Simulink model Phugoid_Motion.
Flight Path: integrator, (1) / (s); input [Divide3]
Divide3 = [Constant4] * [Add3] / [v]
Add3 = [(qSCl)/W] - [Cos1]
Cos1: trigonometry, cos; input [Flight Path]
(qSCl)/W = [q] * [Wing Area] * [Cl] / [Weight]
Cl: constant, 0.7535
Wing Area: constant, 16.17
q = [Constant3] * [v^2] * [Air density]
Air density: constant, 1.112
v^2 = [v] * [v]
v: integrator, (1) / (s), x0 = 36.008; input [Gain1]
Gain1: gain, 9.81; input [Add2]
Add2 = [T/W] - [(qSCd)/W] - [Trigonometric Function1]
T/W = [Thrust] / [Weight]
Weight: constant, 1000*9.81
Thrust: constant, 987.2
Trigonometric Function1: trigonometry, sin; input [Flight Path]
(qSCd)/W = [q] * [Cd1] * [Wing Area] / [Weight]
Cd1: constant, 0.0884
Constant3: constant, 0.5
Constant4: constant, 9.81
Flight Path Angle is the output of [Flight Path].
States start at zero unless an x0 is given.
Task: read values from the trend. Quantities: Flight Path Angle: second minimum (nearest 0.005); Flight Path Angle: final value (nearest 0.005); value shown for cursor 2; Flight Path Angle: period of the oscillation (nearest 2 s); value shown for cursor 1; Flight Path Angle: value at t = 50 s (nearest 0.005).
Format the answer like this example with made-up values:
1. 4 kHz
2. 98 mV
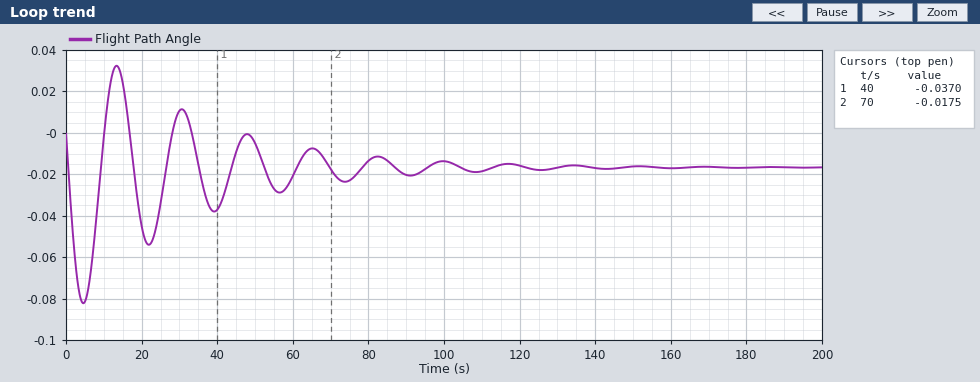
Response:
1. -0.055
2. -0.015
3. -0.0175
4. 18 s
5. -0.0370
6. -0.005
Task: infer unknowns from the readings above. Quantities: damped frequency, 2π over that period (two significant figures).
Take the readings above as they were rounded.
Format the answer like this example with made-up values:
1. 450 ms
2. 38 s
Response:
1. 0.35 rad/s
